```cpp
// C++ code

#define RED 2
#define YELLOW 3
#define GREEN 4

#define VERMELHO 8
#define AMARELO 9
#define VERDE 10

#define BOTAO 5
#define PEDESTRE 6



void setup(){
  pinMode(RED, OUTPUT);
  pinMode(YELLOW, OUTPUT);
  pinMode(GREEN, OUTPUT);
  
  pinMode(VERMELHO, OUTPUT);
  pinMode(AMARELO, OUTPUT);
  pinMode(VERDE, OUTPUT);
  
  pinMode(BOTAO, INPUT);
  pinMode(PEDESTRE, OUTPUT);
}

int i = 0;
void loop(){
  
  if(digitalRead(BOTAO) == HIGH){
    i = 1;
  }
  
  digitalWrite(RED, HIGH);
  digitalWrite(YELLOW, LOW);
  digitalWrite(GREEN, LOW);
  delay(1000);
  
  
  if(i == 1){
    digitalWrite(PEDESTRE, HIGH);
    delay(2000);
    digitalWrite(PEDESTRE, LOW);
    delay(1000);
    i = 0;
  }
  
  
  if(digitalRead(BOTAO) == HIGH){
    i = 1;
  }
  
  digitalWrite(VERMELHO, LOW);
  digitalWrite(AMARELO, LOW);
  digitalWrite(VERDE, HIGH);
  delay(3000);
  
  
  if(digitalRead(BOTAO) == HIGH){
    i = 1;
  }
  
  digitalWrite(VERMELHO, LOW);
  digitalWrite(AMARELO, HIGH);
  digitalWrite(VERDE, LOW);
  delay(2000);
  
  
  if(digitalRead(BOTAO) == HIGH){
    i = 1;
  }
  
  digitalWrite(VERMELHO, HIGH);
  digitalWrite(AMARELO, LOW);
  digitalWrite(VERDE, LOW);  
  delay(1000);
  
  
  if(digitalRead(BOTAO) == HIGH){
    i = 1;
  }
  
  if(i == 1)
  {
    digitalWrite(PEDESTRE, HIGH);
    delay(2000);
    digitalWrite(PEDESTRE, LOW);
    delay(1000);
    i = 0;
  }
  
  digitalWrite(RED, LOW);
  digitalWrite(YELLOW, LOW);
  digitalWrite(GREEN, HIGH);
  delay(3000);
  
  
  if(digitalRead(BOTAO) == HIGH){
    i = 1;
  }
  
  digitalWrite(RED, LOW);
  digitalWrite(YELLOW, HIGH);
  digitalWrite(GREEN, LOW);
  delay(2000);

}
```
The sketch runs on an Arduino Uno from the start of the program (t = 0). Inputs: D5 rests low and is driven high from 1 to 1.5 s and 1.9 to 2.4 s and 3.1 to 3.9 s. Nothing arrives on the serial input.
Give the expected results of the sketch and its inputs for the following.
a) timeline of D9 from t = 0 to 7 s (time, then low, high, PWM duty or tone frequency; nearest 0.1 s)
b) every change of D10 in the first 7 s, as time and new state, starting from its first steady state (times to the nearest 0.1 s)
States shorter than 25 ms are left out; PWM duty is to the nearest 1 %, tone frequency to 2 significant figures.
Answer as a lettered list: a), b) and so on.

a) 0 s low; 4 s high; 6 s low
b) 0 s low; 1 s high; 4 s low
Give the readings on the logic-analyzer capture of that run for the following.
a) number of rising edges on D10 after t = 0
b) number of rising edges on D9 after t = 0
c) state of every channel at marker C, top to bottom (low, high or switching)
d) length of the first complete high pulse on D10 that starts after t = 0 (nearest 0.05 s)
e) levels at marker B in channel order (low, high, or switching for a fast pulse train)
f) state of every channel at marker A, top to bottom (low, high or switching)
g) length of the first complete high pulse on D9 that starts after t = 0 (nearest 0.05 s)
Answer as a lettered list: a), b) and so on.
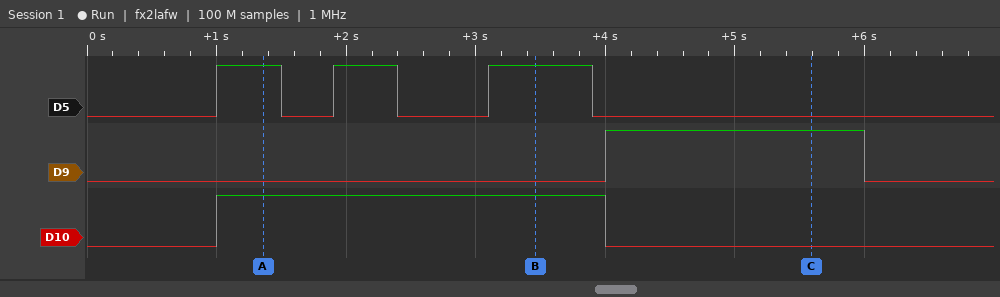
a) 1
b) 1
c) D5 low, D9 high, D10 low
d) 3.00 s
e) D5 high, D9 low, D10 high
f) D5 high, D9 low, D10 high
g) 2.00 s
